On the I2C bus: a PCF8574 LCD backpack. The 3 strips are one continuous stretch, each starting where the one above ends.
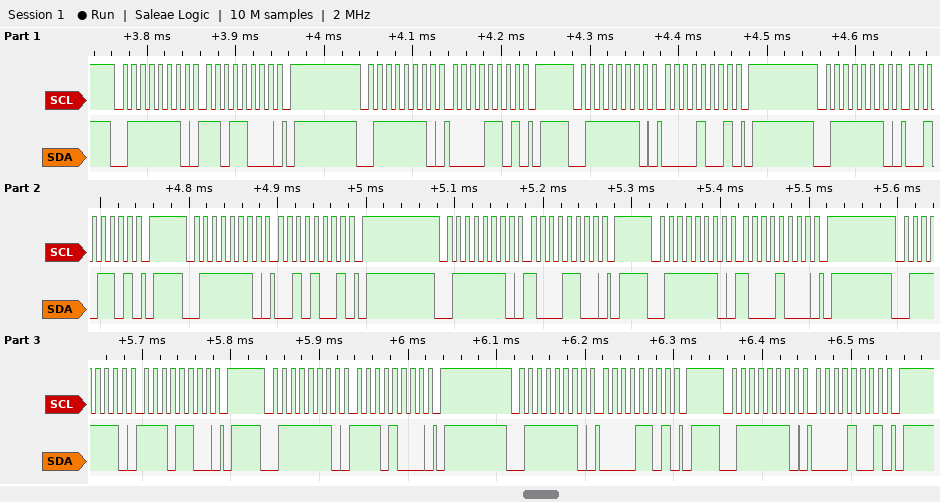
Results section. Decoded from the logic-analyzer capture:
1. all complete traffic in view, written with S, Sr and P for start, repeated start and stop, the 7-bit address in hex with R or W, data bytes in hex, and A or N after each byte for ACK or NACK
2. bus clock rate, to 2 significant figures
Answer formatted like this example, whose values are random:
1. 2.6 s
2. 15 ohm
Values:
1. S 3FW A D8 A P S 3FW A 0D A P S 3FW A 09 A P S 3FW A 2D A P S 3FW A 29 A P S 3FW A 8C A P S 3FW A 88 A P S 3FW A EC A P S 3FW A E8 A P S 3FW A 0D A P S 3FW A 09 A P
2. 100 kHz
